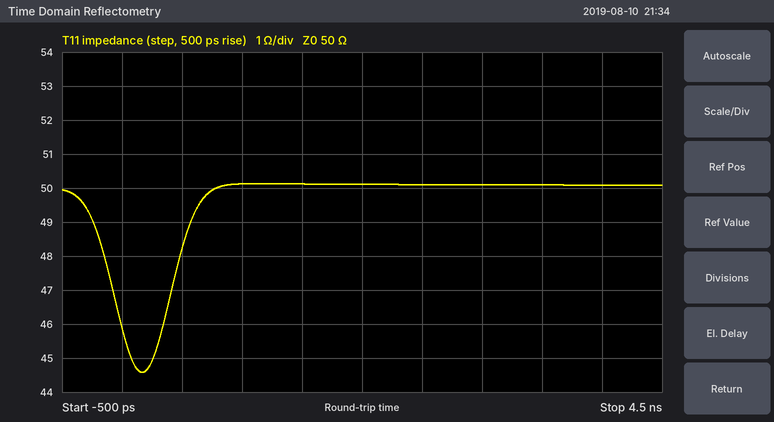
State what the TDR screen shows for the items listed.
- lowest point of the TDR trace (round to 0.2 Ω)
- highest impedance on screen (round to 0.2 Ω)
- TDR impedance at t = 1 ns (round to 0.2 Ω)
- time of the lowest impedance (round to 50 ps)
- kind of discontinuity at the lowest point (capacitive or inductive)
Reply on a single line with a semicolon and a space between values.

44.6 Ω; 50.2 Ω; 50.2 Ω; 150 ps; capacitive
